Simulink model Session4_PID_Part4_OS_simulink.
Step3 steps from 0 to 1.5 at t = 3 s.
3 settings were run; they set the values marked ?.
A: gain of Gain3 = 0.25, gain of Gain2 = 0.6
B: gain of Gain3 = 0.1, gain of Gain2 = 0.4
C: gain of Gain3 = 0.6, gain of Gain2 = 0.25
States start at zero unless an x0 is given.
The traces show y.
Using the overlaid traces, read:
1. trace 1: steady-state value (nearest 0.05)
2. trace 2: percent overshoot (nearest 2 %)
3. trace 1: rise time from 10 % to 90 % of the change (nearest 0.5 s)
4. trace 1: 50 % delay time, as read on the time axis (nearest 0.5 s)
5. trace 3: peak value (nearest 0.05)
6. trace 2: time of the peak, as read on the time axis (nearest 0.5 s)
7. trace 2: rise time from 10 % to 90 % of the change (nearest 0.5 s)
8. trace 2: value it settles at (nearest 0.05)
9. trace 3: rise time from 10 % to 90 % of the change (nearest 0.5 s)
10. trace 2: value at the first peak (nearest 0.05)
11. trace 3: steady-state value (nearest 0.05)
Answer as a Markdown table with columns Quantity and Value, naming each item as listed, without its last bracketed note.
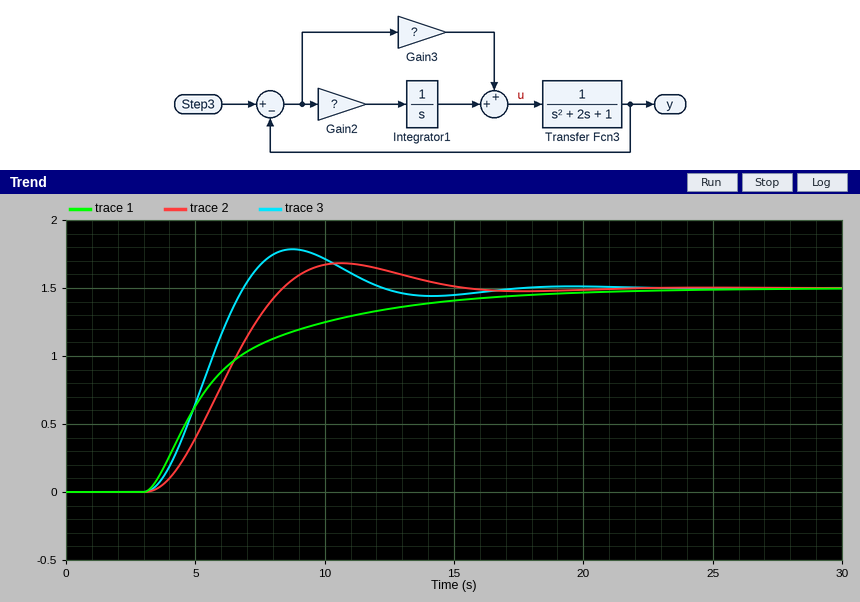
| Quantity | Value |
|---|---|
| trace 1: steady-state value | 1.50 |
| trace 2: percent overshoot | 12 % |
| trace 1: rise time from 10 % to 90 % of the change | 9.0 s |
| trace 1: 50 % delay time, as read on the time axis | 5.5 s |
| trace 3: peak value | 1.80 |
| trace 2: time of the peak, as read on the time axis | 10.5 s |
| trace 2: rise time from 10 % to 90 % of the change | 3.5 s |
| trace 2: value it settles at | 1.50 |
| trace 3: rise time from 10 % to 90 % of the change | 2.5 s |
| trace 2: value at the first peak | 1.70 |
| trace 3: steady-state value | 1.50 |
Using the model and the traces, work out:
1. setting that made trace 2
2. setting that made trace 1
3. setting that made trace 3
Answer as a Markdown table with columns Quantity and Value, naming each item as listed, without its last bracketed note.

| Quantity | Value |
|---|---|
| setting that made trace 2 | B |
| setting that made trace 1 | C |
| setting that made trace 3 | A |
